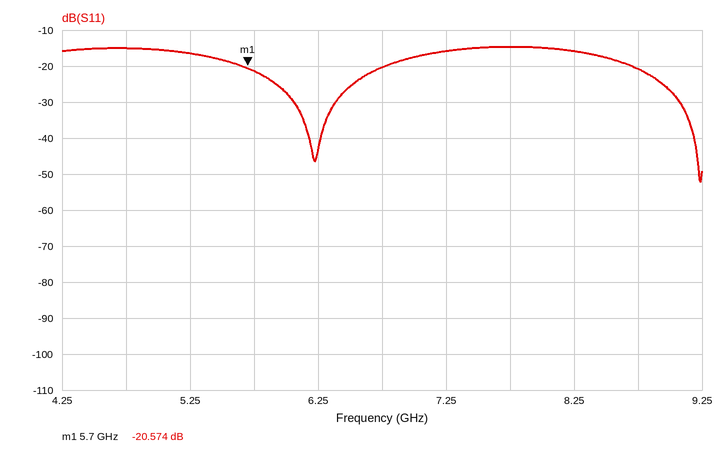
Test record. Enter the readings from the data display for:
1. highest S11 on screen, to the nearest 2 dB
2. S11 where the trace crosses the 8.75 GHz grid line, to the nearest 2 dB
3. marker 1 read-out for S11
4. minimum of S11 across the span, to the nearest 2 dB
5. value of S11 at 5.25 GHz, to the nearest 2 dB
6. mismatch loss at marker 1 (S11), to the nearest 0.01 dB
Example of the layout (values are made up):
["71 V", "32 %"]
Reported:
["-14 dB", "-20 dB", "-20.574 dB", "-52 dB", "-16 dB", "0.04 dB"]
